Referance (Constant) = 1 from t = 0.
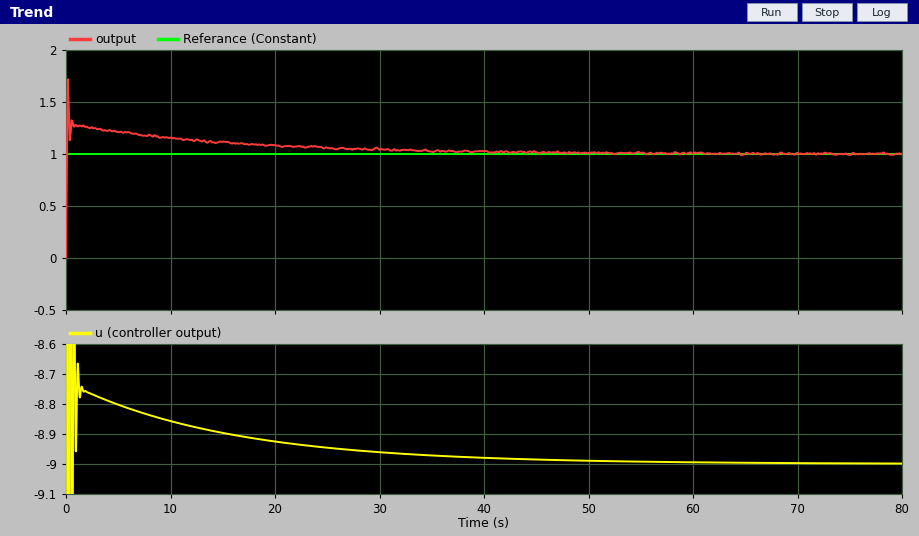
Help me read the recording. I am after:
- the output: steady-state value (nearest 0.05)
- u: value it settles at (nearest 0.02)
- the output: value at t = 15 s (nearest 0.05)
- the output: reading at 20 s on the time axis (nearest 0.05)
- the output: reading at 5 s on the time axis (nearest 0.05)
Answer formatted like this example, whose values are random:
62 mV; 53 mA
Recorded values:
1.00; -9.00; 1.10; 1.10; 1.20
